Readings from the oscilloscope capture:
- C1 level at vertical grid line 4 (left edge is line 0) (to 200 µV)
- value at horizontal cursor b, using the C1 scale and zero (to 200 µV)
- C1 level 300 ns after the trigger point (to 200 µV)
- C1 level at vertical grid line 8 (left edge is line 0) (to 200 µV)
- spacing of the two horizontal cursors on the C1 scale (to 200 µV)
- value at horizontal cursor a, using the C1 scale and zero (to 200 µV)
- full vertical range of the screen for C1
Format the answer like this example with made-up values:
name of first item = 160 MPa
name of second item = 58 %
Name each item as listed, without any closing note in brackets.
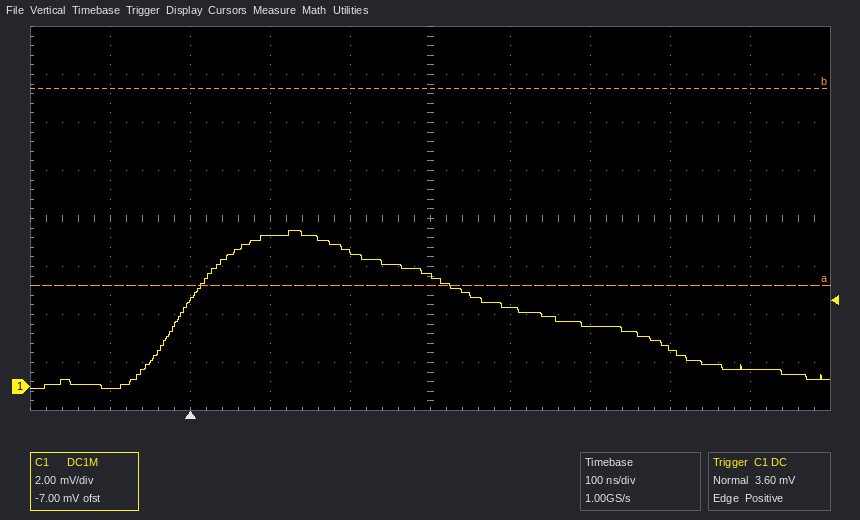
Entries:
C1 level at vertical grid line 4 (left edge is line 0) = 5.6 mV
value at horizontal cursor b, using the C1 scale and zero = 12.4 mV
C1 level 300 ns after the trigger point = 4.6 mV
C1 level at vertical grid line 8 (left edge is line 0) = 1.6 mV
spacing of the two horizontal cursors on the C1 scale = 8.2 mV
value at horizontal cursor a, using the C1 scale and zero = 4.2 mV
full vertical range of the screen for C1 = 16 mV
